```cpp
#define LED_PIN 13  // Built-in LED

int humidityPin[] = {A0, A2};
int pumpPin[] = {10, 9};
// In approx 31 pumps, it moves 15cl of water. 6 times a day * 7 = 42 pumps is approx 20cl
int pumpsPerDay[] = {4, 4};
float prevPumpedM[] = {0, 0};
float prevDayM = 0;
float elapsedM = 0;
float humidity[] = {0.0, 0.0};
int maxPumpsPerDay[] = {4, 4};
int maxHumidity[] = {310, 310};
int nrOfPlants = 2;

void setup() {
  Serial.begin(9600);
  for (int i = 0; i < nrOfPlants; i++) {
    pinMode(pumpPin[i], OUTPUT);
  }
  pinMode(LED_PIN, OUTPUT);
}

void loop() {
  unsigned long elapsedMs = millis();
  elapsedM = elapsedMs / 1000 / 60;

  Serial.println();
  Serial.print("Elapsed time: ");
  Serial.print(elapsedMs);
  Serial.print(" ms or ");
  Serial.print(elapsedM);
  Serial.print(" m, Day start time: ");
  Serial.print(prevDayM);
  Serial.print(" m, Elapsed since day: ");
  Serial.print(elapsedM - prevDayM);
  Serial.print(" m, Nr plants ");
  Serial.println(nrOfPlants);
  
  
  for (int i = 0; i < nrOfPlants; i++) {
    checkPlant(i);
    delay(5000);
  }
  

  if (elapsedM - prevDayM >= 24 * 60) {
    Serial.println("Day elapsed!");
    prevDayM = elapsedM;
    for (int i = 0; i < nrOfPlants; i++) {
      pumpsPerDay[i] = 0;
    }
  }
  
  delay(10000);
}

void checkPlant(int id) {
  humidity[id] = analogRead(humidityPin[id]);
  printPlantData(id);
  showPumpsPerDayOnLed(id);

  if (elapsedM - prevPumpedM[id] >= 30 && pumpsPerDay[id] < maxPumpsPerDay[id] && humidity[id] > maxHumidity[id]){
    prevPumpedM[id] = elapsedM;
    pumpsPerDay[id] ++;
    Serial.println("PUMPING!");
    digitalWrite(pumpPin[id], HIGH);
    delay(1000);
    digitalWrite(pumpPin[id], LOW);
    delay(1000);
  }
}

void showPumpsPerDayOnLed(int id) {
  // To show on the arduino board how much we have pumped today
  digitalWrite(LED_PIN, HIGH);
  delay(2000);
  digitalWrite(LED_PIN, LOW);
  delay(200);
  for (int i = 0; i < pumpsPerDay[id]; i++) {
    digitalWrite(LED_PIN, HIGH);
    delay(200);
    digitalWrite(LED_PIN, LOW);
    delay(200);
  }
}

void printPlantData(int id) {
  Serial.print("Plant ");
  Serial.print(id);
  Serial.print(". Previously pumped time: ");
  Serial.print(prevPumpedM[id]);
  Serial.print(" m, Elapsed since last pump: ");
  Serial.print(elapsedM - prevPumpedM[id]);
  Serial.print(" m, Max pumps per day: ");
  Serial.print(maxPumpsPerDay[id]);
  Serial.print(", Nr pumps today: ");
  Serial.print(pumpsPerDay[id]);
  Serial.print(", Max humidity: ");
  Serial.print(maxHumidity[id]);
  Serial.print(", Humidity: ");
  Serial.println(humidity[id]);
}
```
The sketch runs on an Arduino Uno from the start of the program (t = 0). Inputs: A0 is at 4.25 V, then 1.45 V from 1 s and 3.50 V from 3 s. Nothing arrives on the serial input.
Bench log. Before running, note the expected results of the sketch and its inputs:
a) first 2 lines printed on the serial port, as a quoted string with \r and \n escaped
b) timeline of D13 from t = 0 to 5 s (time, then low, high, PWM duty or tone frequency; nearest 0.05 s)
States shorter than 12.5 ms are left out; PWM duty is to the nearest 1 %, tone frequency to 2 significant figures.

"\r\nElapsed time: 0 ms or 0.00 m, Day start time: 0.00 m, Elapsed since day: 0.00 m, Nr plants 2\r\n"
0 s low; 0.2 s high; 2.2 s low; 2.4 s high; 2.6 s low; 2.8 s high; 3 s low; 3.2 s high; 3.4 s low; 3.6 s high; 3.8 s low
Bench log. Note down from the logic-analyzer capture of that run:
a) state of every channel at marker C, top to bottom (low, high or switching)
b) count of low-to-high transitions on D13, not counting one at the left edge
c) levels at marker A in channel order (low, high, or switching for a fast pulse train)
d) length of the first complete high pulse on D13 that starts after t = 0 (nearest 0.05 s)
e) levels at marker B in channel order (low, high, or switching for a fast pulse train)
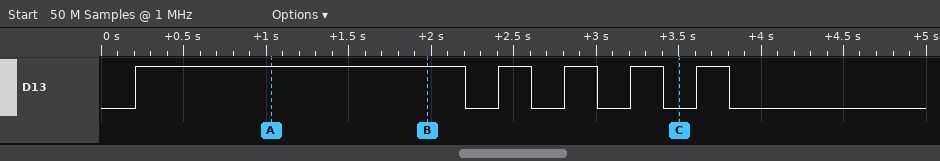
D13 low
5
D13 high
2.00 s
D13 high
